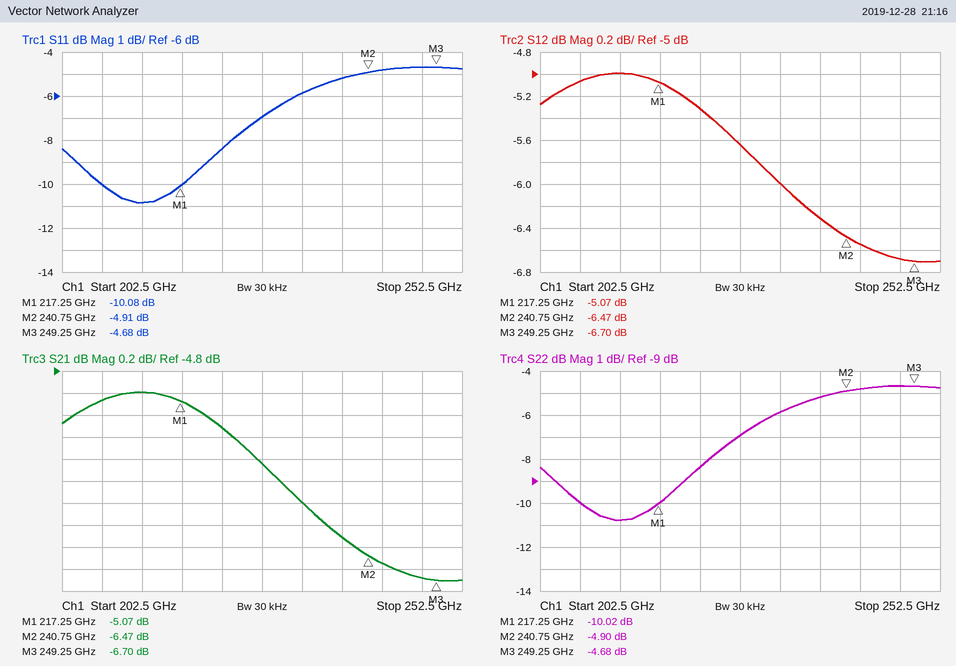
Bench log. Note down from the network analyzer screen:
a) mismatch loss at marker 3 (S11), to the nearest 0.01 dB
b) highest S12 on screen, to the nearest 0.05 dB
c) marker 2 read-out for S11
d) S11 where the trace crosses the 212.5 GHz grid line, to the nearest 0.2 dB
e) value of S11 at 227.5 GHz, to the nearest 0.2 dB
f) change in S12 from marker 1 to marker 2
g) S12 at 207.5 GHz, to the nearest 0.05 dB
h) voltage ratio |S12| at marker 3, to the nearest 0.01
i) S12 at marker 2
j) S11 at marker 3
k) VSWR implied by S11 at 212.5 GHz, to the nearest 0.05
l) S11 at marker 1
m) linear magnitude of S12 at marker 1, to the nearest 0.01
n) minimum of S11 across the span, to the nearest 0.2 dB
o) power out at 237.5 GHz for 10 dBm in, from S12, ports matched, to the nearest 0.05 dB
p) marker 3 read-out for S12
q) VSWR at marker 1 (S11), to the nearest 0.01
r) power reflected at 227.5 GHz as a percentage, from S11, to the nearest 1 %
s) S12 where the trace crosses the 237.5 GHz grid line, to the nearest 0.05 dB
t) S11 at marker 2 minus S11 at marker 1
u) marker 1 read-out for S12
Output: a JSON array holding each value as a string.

["1.81 dB", "-5.00 dB", "-4.91 dB", "-10.8 dB", "-7.0 dB", "-1.40 dB", "-5.05 dB", "0.46", "-6.47 dB", "-4.68 dB", "1.80", "-10.08 dB", "0.56", "-10.8 dB", "3.70 dBm", "-6.70 dB", "1.91", "20 %", "-6.30 dB", "5.17 dB", "-5.07 dB"]
